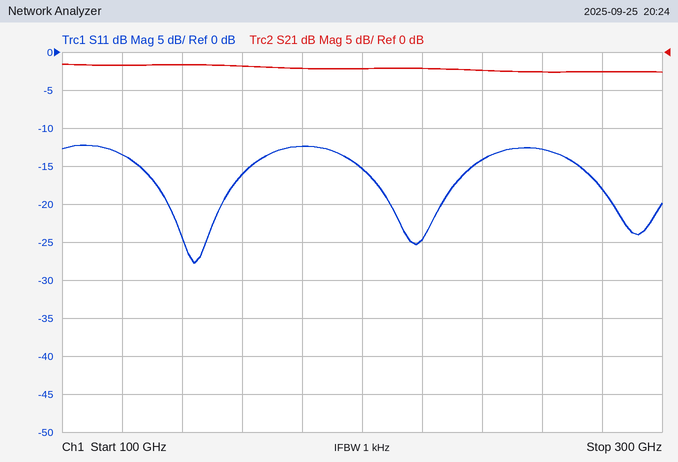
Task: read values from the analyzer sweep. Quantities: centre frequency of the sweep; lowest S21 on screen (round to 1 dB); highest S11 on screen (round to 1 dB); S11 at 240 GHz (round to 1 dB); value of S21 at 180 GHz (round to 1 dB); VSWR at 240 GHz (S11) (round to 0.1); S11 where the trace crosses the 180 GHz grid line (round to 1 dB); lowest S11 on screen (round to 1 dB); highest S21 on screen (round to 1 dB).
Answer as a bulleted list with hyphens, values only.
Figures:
- 200 GHz
- -3 dB
- -12 dB
- -14 dB
- -2 dB
- 1.5
- -12 dB
- -28 dB
- -2 dB
